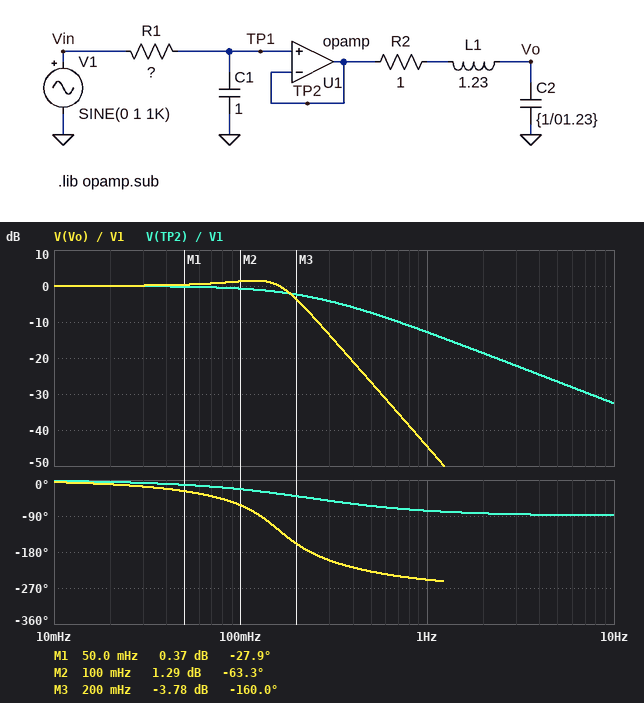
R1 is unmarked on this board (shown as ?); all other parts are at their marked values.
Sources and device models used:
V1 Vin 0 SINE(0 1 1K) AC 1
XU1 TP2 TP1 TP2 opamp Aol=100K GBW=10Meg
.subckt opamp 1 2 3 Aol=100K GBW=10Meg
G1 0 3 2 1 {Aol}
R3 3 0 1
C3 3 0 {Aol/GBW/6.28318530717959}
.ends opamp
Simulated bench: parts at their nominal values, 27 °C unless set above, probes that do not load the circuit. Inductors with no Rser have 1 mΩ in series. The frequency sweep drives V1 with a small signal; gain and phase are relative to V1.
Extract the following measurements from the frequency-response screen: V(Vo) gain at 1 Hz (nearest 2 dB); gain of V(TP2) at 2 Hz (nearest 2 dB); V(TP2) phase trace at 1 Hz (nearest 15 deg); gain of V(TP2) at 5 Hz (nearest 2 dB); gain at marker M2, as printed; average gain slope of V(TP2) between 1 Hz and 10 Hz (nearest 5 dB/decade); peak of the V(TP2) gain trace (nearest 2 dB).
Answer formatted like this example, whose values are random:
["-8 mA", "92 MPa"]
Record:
["-44 dB", "-18 dB", "-75 deg", "-26 dB", "1.29 dB", "-20 dB/decade", "0 dB"]
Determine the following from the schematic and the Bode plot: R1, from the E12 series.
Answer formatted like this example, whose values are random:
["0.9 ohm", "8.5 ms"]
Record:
["0.68 Ω"]
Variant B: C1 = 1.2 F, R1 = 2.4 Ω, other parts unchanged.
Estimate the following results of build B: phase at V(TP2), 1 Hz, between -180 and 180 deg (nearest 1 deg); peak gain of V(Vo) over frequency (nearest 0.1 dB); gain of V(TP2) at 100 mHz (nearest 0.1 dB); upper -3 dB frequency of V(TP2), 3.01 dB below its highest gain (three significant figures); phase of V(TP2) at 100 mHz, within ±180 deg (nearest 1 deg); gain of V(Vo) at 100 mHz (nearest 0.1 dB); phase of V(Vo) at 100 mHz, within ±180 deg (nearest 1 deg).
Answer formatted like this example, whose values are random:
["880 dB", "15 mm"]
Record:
["-87 deg", "0 dB", "-6.3 dB", "55.3 mHz", "-61 deg", "-4.3 dB", "-101 deg"]
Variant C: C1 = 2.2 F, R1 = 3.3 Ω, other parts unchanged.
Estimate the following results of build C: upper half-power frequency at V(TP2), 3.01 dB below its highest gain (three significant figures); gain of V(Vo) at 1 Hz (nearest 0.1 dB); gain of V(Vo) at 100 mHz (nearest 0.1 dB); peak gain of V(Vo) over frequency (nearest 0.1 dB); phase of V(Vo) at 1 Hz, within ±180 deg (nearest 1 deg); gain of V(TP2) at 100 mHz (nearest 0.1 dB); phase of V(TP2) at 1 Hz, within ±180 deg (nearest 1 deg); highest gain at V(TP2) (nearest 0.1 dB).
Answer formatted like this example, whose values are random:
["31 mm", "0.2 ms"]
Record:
["21.9 mHz", "-65.0 dB", "-11.4 dB", "0 dB", "99 deg", "-13.4 dB", "-89 deg", "0 dB"]
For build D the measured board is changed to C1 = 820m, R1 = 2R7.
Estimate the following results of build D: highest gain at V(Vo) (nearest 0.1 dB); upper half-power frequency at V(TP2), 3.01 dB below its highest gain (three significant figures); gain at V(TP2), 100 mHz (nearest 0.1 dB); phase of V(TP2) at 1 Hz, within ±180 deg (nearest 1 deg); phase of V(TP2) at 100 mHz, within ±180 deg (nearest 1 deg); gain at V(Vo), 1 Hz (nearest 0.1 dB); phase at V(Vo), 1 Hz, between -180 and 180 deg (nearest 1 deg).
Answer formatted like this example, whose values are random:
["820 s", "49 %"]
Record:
["0 dB", "71.9 mHz", "-4.7 dB", "-86 deg", "-54 deg", "-54.7 dB", "102 deg"]
